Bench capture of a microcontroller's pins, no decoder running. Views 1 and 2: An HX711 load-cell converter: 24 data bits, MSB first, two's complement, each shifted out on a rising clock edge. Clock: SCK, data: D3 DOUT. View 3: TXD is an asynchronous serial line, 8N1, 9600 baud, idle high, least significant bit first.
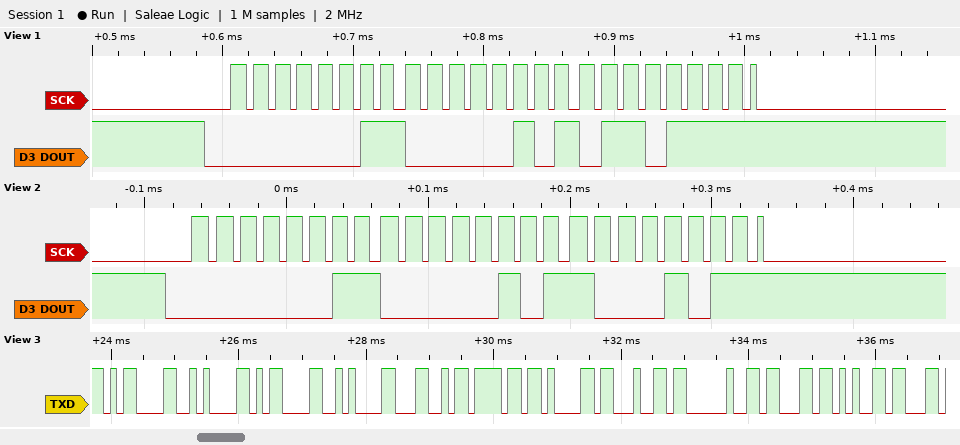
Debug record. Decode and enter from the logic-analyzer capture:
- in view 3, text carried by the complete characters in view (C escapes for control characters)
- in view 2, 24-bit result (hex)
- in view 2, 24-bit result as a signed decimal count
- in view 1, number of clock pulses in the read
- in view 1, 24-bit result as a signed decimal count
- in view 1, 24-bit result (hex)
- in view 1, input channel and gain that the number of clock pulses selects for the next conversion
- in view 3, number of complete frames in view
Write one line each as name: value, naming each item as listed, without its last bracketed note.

in view 3, text carried by the complete characters in view: "\r\n\r\nLoad ce"
in view 2, 24-bit result: 0x03058B
in view 2, 24-bit result as a signed decimal count: 198027
in view 1, number of clock pulses in the read: 25
in view 1, 24-bit result as a signed decimal count: 197999
in view 1, 24-bit result: 0x03056F
in view 1, input channel and gain that the number of clock pulses selects for the next conversion: channel A, gain 128
in view 3, number of complete frames in view: 11
